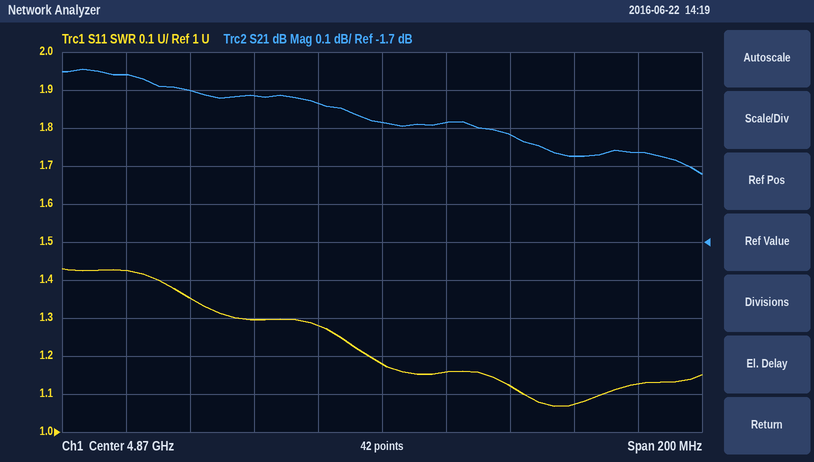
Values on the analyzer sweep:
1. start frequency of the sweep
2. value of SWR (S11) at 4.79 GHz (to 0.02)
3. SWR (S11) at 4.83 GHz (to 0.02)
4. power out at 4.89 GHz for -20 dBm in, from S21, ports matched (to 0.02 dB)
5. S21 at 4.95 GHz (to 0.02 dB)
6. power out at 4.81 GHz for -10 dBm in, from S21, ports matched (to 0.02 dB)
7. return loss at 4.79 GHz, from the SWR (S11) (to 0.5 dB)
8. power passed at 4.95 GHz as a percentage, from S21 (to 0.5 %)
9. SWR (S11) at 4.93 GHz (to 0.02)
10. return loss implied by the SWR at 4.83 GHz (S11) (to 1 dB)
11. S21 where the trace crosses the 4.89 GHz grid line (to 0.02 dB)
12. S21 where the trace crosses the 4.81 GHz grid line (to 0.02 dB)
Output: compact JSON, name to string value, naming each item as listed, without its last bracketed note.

{"start frequency of the sweep": "4.77 GHz", "value of SWR (S11) at 4.79 GHz": "1.42", "SWR (S11) at 4.83 GHz": "1.30", "power out at 4.89 GHz for -20 dBm in, from S21, ports matched": "-21.38 dBm", "S21 at 4.95 GHz": "-1.46 dB", "power out at 4.81 GHz for -10 dBm in, from S21, ports matched": "-11.30 dBm", "return loss at 4.79 GHz, from the SWR (S11)": "15.0 dB", "power passed at 4.95 GHz as a percentage, from S21": "71.5 %", "SWR (S11) at 4.93 GHz": "1.08", "return loss implied by the SWR at 4.83 GHz (S11)": "18 dB", "S21 where the trace crosses the 4.89 GHz grid line": "-1.38 dB", "S21 where the trace crosses the 4.81 GHz grid line": "-1.30 dB"}
